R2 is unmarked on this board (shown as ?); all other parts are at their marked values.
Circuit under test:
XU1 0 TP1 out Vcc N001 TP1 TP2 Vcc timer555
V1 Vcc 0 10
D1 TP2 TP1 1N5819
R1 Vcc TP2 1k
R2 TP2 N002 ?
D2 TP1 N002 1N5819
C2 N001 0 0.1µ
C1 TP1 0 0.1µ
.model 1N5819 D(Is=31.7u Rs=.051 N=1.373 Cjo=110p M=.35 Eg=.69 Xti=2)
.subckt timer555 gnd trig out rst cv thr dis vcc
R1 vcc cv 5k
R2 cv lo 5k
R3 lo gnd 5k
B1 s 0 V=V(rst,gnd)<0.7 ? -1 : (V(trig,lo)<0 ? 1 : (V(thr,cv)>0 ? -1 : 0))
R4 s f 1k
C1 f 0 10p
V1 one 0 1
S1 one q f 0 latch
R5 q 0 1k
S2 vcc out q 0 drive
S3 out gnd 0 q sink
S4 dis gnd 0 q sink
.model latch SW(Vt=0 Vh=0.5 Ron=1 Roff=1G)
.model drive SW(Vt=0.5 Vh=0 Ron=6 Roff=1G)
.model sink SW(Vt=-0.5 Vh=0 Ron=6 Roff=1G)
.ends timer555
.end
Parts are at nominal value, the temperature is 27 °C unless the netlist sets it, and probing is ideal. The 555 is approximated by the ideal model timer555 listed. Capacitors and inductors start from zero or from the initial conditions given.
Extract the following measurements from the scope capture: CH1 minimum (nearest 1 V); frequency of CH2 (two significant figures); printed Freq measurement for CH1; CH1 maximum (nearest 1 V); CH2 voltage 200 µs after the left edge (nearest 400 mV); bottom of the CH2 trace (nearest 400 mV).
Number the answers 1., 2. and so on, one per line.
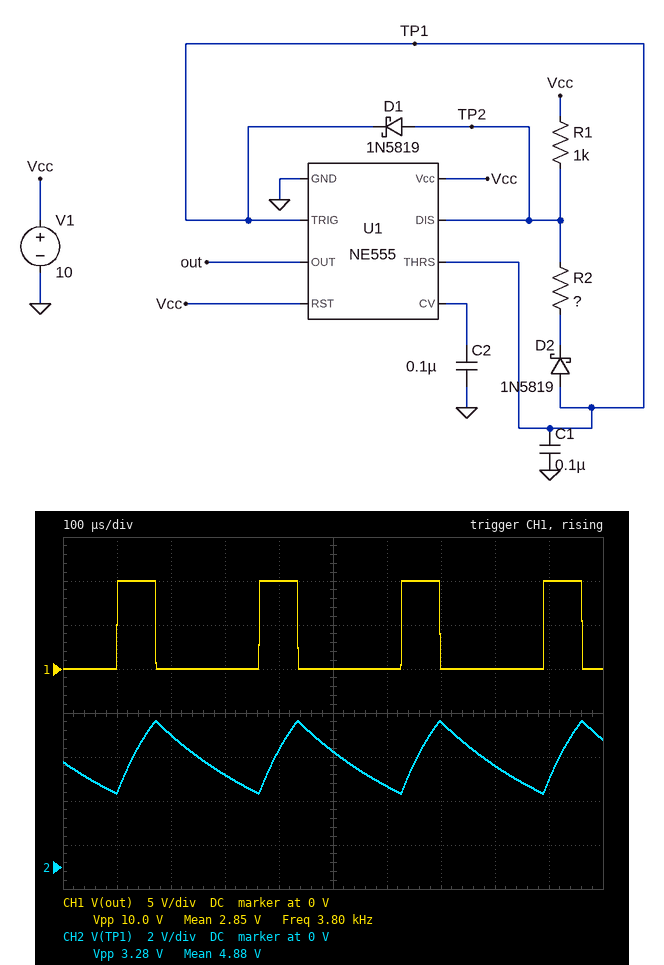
1. 0 V
2. 3.8 kHz
3. 3.80 kHz
4. 10 V
5. 6.0 V
6. 3.2 V
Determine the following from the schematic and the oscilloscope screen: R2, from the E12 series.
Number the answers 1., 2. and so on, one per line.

1. 2.7 kΩ
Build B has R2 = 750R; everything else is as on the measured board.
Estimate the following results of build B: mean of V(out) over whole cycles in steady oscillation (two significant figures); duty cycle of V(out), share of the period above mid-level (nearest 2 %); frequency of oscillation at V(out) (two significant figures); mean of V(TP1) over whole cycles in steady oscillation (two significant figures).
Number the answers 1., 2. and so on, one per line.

1. 5.7 V
2. 56 %
3. 7.9 kHz
4. 5.0 V
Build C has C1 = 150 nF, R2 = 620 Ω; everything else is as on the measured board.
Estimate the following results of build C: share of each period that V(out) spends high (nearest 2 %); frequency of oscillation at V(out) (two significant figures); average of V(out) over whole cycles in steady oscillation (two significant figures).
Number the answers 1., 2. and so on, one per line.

1. 62 %
2. 5.7 kHz
3. 6.1 V
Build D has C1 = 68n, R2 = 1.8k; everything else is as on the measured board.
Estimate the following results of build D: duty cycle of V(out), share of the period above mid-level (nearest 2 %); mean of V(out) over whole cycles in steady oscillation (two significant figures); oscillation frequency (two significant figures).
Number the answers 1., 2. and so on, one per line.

1. 36 %
2. 3.6 V
3. 7.3 kHz
